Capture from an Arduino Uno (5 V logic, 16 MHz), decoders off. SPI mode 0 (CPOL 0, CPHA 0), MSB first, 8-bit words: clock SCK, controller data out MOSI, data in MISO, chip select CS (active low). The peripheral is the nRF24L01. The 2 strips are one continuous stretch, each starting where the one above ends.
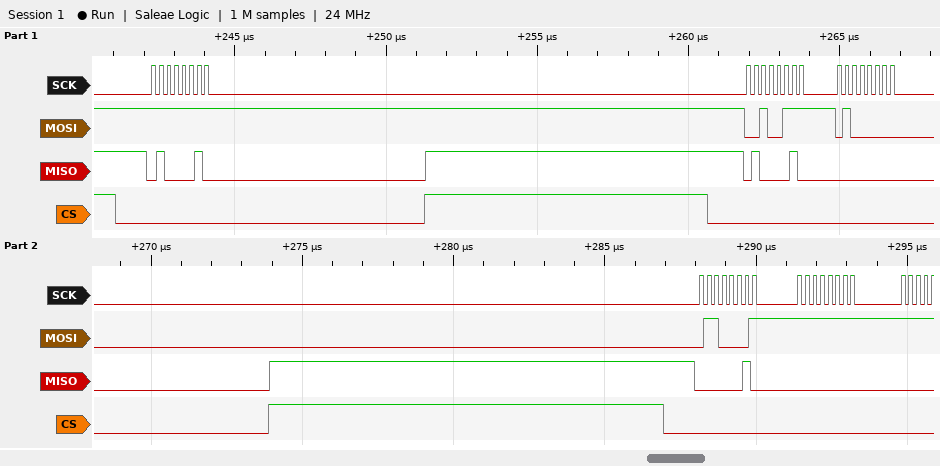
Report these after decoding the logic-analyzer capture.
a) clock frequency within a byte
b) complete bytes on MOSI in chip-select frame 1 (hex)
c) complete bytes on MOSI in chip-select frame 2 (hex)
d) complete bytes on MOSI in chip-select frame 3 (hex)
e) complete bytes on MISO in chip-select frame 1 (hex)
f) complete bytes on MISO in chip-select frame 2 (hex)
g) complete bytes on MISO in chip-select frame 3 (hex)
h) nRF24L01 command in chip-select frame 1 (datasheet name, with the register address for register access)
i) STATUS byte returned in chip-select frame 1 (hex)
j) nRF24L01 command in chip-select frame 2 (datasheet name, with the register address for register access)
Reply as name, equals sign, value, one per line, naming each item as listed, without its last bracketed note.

clock frequency within a byte = 4 MHz
complete bytes on MOSI in chip-select frame 1 = FF
complete bytes on MOSI in chip-select frame 2 = 27 40
complete bytes on MOSI in chip-select frame 3 = 61 FF
complete bytes on MISO in chip-select frame 1 = 42
complete bytes on MISO in chip-select frame 2 = 42 00
complete bytes on MISO in chip-select frame 3 = 02 00
nRF24L01 command in chip-select frame 1 = NOP
STATUS byte returned in chip-select frame 1 = 0x42
nRF24L01 command in chip-select frame 2 = W_REGISTER 0x07
